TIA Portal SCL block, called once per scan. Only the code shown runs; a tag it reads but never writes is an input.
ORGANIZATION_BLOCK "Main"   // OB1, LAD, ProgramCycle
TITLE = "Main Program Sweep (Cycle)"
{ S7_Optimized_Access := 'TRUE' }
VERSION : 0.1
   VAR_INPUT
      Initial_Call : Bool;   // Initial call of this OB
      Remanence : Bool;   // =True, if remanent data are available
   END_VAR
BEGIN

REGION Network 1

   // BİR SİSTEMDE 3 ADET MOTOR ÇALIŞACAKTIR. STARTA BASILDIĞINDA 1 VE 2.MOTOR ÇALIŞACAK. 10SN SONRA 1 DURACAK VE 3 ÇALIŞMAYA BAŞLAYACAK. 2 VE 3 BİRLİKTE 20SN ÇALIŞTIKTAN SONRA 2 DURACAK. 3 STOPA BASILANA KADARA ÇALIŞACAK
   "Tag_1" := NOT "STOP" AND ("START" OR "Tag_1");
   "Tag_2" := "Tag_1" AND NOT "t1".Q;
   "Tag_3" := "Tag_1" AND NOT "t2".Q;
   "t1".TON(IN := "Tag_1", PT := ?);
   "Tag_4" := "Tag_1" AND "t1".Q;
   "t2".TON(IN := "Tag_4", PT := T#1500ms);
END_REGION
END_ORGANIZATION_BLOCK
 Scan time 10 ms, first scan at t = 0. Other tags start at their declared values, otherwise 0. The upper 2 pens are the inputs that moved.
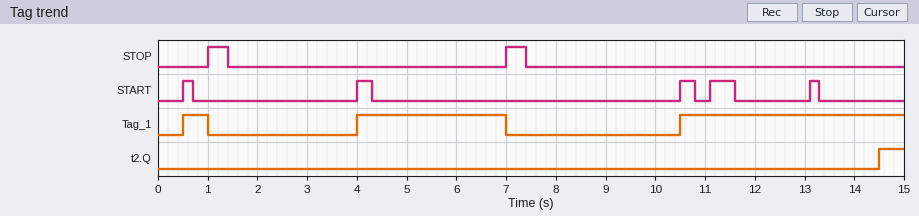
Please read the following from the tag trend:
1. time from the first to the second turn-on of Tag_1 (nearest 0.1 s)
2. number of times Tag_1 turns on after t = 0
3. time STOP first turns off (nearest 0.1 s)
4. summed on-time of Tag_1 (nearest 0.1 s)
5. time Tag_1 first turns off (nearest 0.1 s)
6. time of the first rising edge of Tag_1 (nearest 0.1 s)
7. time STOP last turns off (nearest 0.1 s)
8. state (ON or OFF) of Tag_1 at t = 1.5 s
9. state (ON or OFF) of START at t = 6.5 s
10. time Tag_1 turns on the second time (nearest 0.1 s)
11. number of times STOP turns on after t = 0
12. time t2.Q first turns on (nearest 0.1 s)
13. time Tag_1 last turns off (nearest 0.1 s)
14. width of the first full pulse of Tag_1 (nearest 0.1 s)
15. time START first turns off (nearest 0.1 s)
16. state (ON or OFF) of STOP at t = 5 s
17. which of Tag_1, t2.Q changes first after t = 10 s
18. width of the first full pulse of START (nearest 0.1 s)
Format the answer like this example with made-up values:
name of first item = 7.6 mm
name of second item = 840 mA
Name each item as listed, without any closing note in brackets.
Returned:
time from the first to the second turn-on of Tag_1 = 3.5 s
number of times Tag_1 turns on after t = 0 = 3
time STOP first turns off = 1.4 s
summed on-time of Tag_1 = 8.0 s
time Tag_1 first turns off = 1.0 s
time of the first rising edge of Tag_1 = 0.5 s
time STOP last turns off = 7.4 s
state (ON or OFF) of Tag_1 at t = 1.5 s = OFF
state (ON or OFF) of START at t = 6.5 s = OFF
time Tag_1 turns on the second time = 4.0 s
number of times STOP turns on after t = 0 = 2
time t2.Q first turns on = 14.5 s
time Tag_1 last turns off = 7.0 s
width of the first full pulse of Tag_1 = 0.5 s
time START first turns off = 0.7 s
state (ON or OFF) of STOP at t = 5 s = OFF
which of Tag_1, t2.Q changes first after t = 10 s = Tag_1
width of the first full pulse of START = 0.2 s
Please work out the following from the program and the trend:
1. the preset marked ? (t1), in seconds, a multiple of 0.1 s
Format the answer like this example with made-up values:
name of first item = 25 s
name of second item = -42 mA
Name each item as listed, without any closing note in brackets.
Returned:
the preset marked ? (t1), in seconds, a multiple of 0.1 s = 2.5 s
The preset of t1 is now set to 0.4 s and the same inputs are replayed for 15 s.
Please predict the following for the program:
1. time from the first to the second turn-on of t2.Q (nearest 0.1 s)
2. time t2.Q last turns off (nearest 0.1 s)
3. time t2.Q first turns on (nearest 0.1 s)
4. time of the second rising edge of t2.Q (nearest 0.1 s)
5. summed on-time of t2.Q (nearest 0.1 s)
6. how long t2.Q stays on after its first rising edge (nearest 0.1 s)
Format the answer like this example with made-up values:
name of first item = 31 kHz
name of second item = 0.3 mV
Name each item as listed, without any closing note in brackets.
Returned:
time from the first to the second turn-on of t2.Q = 6.5 s
time t2.Q last turns off = 7.0 s
time t2.Q first turns on = 5.9 s
time of the second rising edge of t2.Q = 12.4 s
summed on-time of t2.Q = 3.7 s
how long t2.Q stays on after its first rising edge = 1.1 s
